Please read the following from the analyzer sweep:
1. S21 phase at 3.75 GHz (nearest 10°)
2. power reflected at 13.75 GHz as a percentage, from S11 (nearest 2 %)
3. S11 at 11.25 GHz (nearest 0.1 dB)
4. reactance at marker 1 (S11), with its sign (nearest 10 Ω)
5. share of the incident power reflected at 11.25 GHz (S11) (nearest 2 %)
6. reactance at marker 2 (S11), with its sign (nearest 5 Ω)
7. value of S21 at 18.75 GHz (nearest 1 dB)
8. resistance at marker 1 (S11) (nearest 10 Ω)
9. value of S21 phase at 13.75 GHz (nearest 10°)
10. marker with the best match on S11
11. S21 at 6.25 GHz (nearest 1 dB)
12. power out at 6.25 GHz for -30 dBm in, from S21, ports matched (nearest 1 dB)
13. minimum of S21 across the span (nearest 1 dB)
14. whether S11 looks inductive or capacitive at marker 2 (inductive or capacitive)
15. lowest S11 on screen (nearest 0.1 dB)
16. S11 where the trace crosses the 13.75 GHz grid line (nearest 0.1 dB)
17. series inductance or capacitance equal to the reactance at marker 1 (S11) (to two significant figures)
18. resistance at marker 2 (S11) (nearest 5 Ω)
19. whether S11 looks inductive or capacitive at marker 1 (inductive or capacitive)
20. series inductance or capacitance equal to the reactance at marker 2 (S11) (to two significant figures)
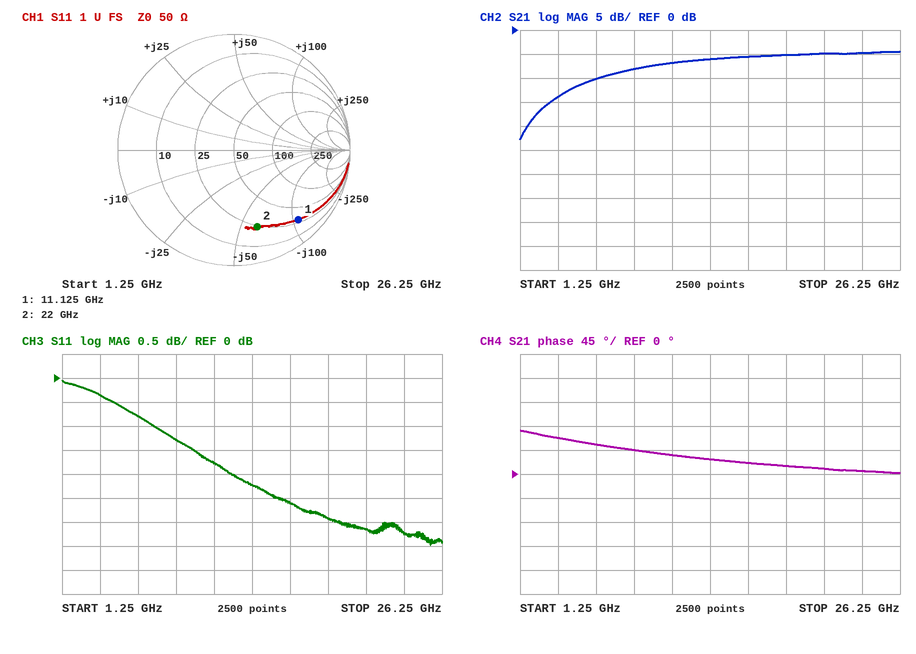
70°
60 %
-1.8 dB
-110 Ω
66 %
-60 Ω
-5 dB
30 Ω
30°
marker 2
-10 dB
-40 dBm
-23 dB
capacitive
-3.5 dB
-2.2 dB
130 fF
25 Ω
capacitive
120 fF
